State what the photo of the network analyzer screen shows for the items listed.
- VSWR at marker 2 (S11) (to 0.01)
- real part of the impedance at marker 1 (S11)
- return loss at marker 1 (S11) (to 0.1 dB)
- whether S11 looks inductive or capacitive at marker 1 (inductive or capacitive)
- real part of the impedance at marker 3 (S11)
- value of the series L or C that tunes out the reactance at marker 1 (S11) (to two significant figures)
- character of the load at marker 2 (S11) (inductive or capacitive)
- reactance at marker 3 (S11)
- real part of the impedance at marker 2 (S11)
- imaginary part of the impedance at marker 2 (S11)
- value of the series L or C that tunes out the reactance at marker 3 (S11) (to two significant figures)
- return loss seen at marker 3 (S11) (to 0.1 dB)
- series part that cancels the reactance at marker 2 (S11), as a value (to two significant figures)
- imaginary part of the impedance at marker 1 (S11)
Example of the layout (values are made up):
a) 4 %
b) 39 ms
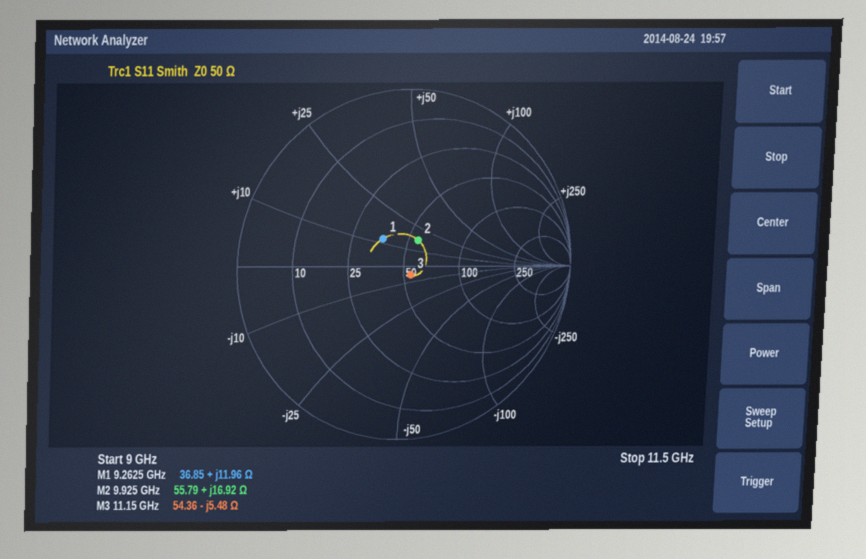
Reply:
a) 1.40
b) 36.85 Ω
c) 13.9 dB
d) inductive
e) 54.36 Ω
f) 1.4 pF
g) inductive
h) -5.48 Ω
i) 55.79 Ω
j) +16.92 Ω
k) 78 pH
l) 23.5 dB
m) 950 fF
n) +11.96 Ω
